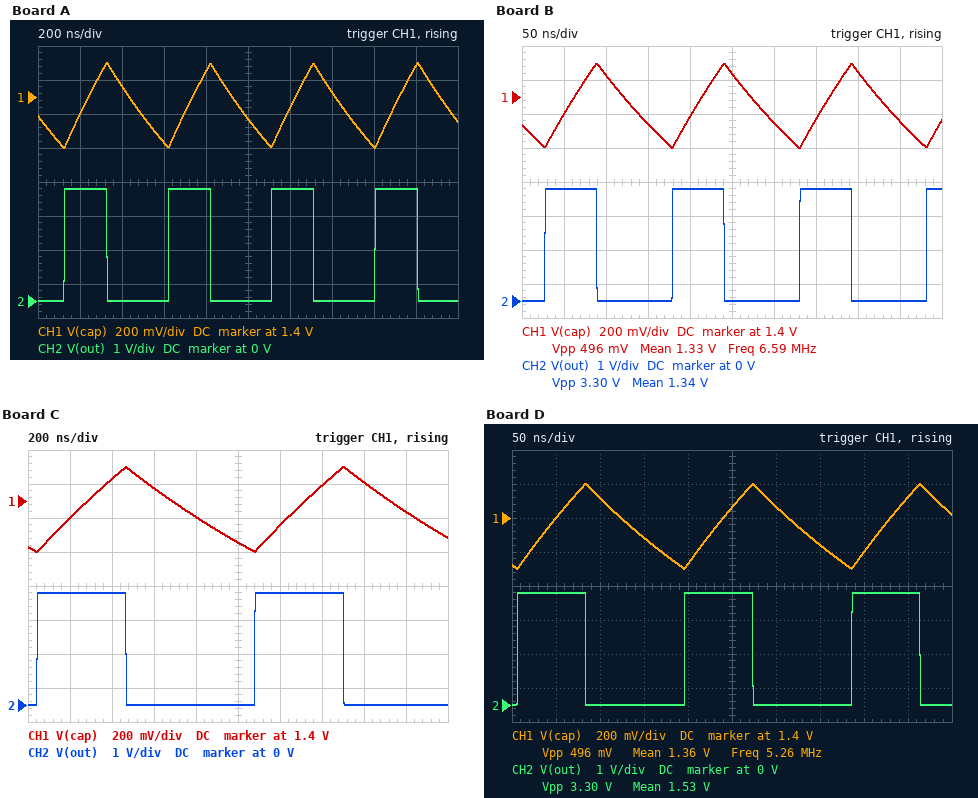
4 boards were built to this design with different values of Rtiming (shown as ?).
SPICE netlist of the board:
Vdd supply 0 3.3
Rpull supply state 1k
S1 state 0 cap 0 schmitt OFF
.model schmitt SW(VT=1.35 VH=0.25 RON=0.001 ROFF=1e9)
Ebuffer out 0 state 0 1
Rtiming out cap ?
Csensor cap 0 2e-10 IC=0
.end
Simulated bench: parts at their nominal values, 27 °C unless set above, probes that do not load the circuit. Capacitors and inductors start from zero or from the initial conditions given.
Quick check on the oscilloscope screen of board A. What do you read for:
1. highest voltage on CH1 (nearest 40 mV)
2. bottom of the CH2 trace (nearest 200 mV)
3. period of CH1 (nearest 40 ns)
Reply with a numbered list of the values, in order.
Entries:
1. 1.60 V
2. 0 V
3. 480 ns
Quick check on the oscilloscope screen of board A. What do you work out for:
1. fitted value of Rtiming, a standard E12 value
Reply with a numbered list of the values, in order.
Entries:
1. 3.9 kΩ
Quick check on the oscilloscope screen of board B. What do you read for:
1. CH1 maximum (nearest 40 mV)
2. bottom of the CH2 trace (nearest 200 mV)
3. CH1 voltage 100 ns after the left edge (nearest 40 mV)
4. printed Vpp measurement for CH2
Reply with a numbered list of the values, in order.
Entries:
1. 1.60 V
2. 0 V
3. 1.52 V
4. 3.30 V
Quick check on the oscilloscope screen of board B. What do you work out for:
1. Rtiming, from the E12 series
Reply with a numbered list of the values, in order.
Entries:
1. 1.2 kΩ
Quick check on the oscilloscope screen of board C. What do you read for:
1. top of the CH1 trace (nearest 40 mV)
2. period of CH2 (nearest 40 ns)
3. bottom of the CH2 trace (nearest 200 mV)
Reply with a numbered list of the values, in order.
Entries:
1. 1.60 V
2. 1.04 µs
3. 0 V
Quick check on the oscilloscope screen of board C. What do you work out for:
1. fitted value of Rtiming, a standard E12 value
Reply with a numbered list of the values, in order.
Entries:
1. 8.2 kΩ
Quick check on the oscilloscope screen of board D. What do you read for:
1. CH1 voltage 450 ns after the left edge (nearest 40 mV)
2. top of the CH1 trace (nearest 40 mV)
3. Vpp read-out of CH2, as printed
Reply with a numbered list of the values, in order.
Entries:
1. 1.52 V
2. 1.60 V
3. 3.30 V
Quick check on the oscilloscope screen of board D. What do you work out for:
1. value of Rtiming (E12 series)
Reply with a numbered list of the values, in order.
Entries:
1. 1.5 kΩ
